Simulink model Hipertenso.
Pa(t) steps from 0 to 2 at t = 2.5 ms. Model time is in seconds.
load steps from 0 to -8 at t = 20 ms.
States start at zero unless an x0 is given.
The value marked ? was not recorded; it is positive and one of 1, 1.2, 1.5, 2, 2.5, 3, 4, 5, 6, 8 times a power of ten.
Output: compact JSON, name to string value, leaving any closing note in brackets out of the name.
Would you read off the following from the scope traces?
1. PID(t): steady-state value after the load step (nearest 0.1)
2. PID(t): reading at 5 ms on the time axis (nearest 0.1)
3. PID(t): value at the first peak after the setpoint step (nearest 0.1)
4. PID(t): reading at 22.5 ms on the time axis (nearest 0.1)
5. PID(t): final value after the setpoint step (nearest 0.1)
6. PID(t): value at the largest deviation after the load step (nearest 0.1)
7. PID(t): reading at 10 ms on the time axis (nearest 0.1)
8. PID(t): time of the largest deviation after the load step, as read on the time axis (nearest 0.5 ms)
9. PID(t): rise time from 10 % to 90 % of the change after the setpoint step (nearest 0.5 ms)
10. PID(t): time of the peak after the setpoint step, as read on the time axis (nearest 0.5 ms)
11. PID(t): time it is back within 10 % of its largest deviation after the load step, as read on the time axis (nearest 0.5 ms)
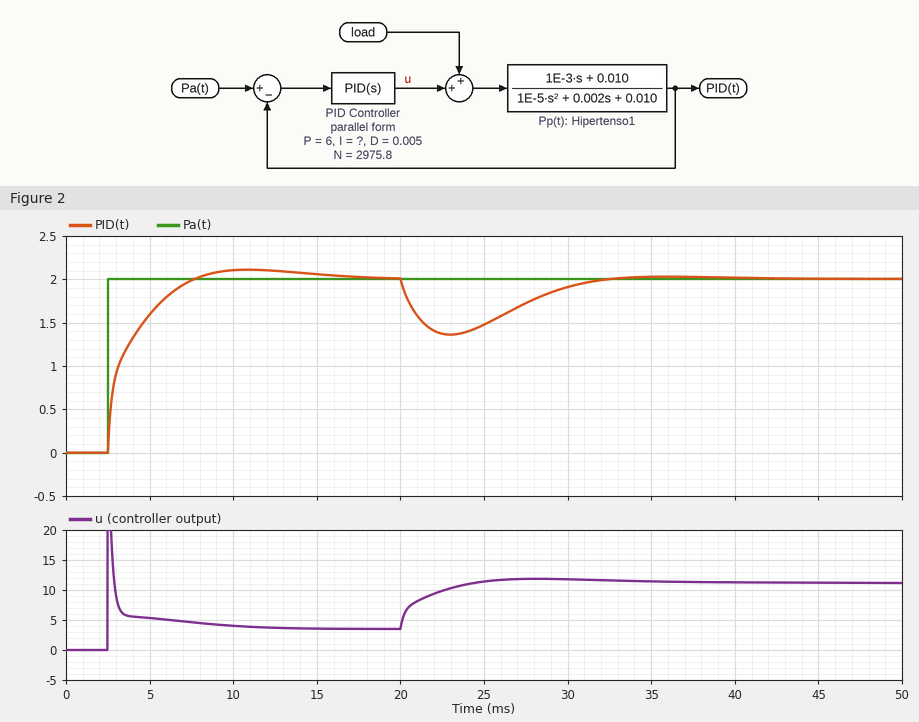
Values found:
{"PID(t): steady-state value after the load step": "2.0", "PID(t): reading at 5 ms on the time axis": "1.6", "PID(t): value at the first peak after the setpoint step": "2.1", "PID(t): reading at 22.5 ms on the time axis": "1.4", "PID(t): final value after the setpoint step": "2.0", "PID(t): value at the largest deviation after the load step": "1.4", "PID(t): reading at 10 ms on the time axis": "2.1", "PID(t): time of the largest deviation after the load step, as read on the time axis": "23.0 ms", "PID(t): rise time from 10 % to 90 % of the change after the setpoint step": "3.5 ms", "PID(t): time of the peak after the setpoint step, as read on the time axis": "11.0 ms", "PID(t): time it is back within 10 % of its largest deviation after the load step, as read on the time axis": "30.5 ms"}
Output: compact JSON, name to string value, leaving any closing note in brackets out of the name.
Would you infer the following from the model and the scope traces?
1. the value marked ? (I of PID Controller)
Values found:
{"the value marked ?": "2000"}
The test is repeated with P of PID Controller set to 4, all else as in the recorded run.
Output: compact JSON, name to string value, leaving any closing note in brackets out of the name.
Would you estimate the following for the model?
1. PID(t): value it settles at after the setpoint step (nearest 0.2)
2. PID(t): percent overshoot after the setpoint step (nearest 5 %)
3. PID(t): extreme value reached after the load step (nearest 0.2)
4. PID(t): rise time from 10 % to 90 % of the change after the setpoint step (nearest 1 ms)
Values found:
{"PID(t): value it settles at after the setpoint step": "2.0", "PID(t): percent overshoot after the setpoint step": "10 %", "PID(t): extreme value reached after the load step": "1.2", "PID(t): rise time from 10 % to 90 % of the change after the setpoint step": "4 ms"}
